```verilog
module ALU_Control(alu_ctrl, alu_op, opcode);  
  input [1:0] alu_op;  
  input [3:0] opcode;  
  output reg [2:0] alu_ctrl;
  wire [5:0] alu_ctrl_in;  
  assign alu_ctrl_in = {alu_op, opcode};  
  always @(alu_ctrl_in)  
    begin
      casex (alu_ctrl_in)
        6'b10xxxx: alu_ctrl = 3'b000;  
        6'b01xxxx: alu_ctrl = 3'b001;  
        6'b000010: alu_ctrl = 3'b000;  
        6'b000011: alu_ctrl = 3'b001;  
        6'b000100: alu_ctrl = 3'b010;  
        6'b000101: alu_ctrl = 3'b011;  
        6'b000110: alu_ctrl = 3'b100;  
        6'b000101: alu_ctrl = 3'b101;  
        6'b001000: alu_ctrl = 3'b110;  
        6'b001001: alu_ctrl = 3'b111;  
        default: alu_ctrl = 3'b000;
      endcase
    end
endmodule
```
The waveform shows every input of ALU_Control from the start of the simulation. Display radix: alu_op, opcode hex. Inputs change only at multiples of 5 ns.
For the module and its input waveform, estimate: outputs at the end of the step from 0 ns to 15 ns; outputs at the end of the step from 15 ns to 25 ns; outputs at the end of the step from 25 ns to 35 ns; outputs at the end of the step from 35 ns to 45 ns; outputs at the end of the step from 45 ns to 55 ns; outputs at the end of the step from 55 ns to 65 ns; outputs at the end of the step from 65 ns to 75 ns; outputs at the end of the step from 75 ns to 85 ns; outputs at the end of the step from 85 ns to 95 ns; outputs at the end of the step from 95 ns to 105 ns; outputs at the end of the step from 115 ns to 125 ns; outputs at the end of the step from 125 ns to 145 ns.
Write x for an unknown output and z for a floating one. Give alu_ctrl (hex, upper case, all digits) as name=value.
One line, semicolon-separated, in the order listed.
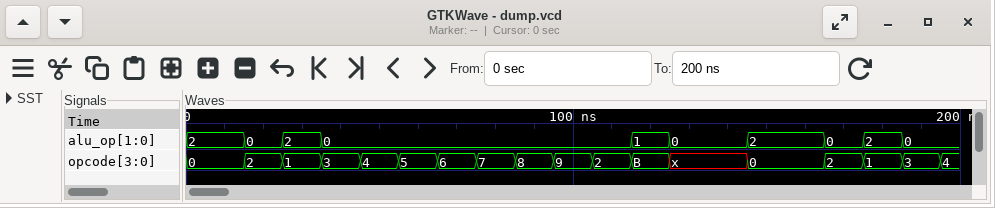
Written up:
alu_ctrl=0; alu_ctrl=0; alu_ctrl=0; alu_ctrl=1; alu_ctrl=2; alu_ctrl=3; alu_ctrl=4; alu_ctrl=0; alu_ctrl=6; alu_ctrl=7; alu_ctrl=1; alu_ctrl=0
